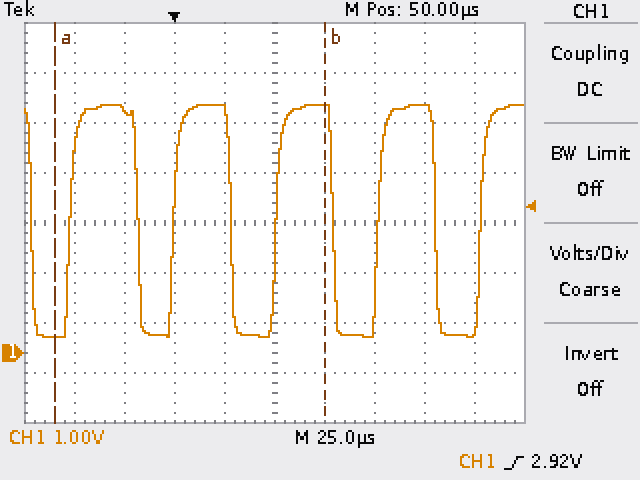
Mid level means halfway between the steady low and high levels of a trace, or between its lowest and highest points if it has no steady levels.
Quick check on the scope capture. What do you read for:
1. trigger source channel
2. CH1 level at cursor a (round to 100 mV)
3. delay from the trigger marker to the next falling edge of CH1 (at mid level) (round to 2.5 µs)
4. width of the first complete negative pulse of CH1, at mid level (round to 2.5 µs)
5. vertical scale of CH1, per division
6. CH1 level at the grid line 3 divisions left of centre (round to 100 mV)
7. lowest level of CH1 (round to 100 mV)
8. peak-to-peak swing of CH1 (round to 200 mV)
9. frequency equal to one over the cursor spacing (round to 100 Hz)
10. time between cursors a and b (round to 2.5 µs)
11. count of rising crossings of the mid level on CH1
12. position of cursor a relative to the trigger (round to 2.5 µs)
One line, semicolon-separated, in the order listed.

CH1; 300 mV; 27.5 µs; 20.0 µs; 1 V; 4.9 V; 300 mV; 4.6 V; 7.4 kHz; 135.0 µs; 5; -60.0 µs
